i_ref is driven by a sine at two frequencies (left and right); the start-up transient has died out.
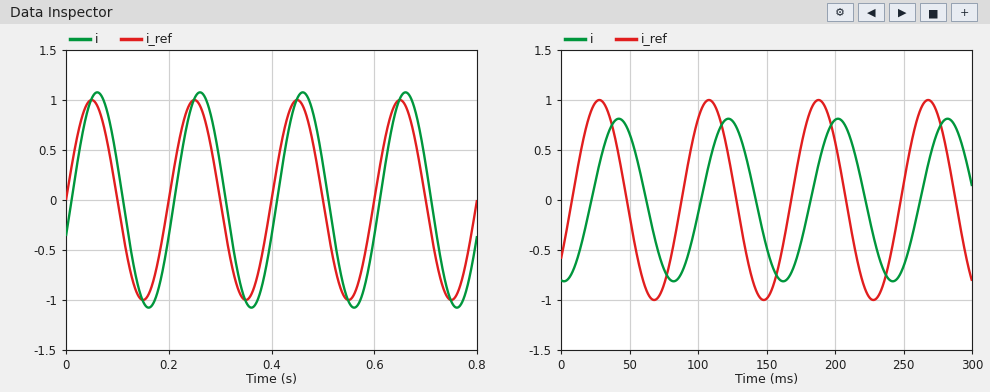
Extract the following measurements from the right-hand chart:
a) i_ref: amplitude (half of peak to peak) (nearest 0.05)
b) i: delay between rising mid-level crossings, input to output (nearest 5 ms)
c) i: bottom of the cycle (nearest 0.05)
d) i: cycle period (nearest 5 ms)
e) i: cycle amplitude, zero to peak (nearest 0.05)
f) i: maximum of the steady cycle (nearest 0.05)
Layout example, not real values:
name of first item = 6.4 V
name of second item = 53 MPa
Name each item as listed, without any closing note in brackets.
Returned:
i_ref: amplitude (half of peak to peak) = 1.00
i: delay between rising mid-level crossings, input to output = 15 ms
i: bottom of the cycle = -0.80
i: cycle period = 80 ms
i: cycle amplitude, zero to peak = 0.80
i: maximum of the steady cycle = 0.80
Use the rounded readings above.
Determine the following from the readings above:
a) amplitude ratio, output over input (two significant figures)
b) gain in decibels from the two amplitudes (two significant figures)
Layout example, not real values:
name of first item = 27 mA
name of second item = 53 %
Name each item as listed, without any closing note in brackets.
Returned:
amplitude ratio, output over input = 0.80
gain in decibels from the two amplitudes = -1.9 dB
